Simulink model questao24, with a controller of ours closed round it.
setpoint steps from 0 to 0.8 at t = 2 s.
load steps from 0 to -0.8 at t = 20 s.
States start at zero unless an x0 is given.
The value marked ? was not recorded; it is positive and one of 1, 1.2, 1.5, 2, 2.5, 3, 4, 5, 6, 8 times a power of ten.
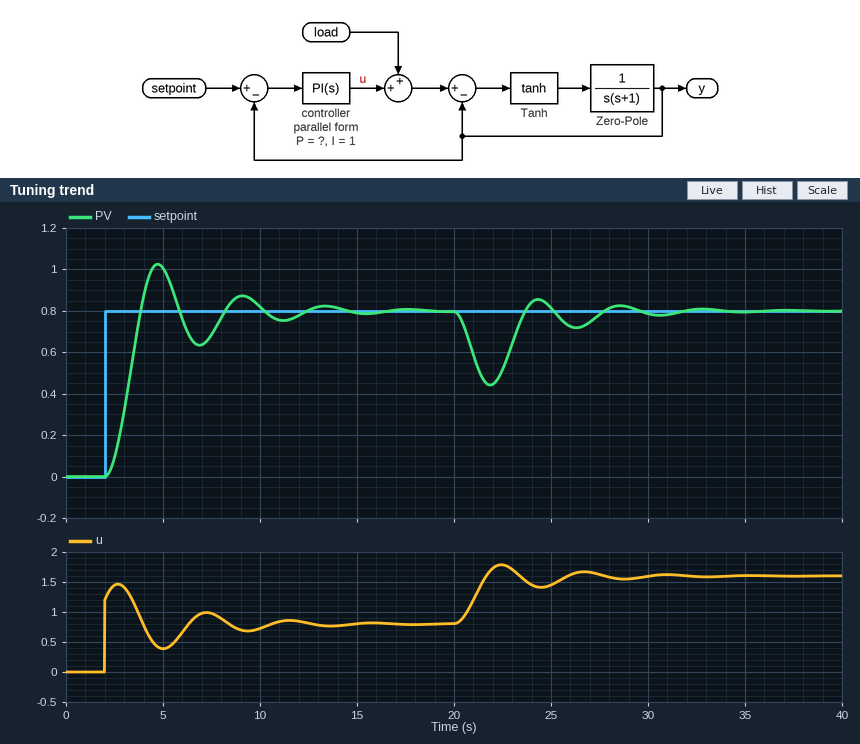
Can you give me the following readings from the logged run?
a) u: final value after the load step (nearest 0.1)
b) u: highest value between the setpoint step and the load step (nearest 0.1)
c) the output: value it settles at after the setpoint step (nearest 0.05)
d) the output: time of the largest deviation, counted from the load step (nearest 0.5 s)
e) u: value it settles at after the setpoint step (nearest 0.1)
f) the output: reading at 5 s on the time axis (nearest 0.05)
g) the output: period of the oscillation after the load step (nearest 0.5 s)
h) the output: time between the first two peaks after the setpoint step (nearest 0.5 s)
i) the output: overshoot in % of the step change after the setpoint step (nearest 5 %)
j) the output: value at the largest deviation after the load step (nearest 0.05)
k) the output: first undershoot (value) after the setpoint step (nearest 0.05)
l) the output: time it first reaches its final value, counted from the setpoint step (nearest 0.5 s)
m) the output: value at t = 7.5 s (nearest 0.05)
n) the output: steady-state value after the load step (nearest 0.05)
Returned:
1.6
1.5
0.80
2.0 s
0.8
1.00
4.5 s
4.5 s
30 %
0.45
0.65
2.0 s
0.70
0.80
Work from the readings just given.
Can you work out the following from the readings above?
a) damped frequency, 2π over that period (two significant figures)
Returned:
1.4 rad/s
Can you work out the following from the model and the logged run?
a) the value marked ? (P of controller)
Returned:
1.5
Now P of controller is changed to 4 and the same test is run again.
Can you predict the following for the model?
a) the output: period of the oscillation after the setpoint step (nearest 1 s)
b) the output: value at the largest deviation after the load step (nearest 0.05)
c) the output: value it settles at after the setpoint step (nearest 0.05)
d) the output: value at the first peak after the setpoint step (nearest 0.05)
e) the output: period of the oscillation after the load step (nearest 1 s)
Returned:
3 s
0.60
0.80
1.00
3 s
